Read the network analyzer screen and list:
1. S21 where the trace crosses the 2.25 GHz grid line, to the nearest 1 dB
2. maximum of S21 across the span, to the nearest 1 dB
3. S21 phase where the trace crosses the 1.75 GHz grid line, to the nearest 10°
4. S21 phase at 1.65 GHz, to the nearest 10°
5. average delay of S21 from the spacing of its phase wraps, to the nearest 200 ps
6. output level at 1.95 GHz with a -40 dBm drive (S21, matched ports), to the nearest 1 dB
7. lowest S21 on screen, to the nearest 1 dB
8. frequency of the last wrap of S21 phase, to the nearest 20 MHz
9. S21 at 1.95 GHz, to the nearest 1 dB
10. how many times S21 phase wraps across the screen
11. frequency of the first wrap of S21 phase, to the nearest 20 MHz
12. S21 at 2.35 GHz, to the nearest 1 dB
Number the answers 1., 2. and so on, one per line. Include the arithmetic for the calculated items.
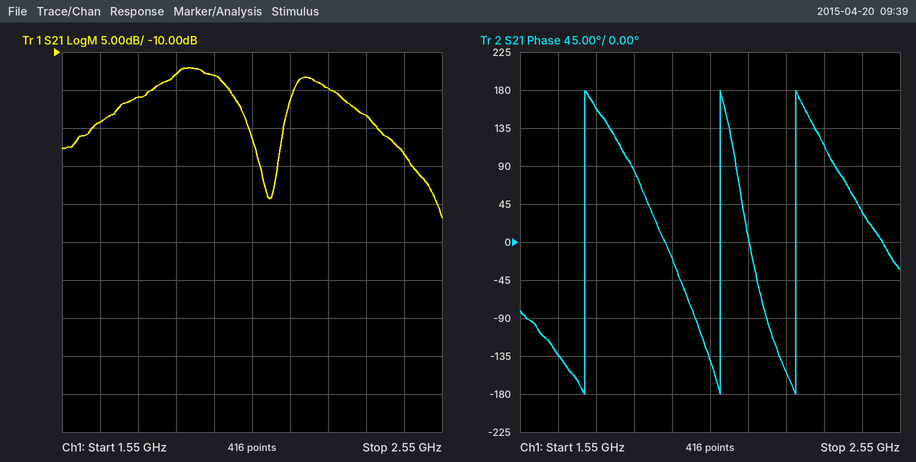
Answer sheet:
1. -15 dB
2. -12 dB
3. 160°
4. -130°
5. 2 cycles / (2.28 GHz − 1.72 GHz) ≈ 3.6 ns
6. -40 dBm + (-13 dB) = -53 dBm
7. -32 dB
8. 2.28 GHz
9. -13 dB
10. 3
11. 1.72 GHz
12. -18 dB
